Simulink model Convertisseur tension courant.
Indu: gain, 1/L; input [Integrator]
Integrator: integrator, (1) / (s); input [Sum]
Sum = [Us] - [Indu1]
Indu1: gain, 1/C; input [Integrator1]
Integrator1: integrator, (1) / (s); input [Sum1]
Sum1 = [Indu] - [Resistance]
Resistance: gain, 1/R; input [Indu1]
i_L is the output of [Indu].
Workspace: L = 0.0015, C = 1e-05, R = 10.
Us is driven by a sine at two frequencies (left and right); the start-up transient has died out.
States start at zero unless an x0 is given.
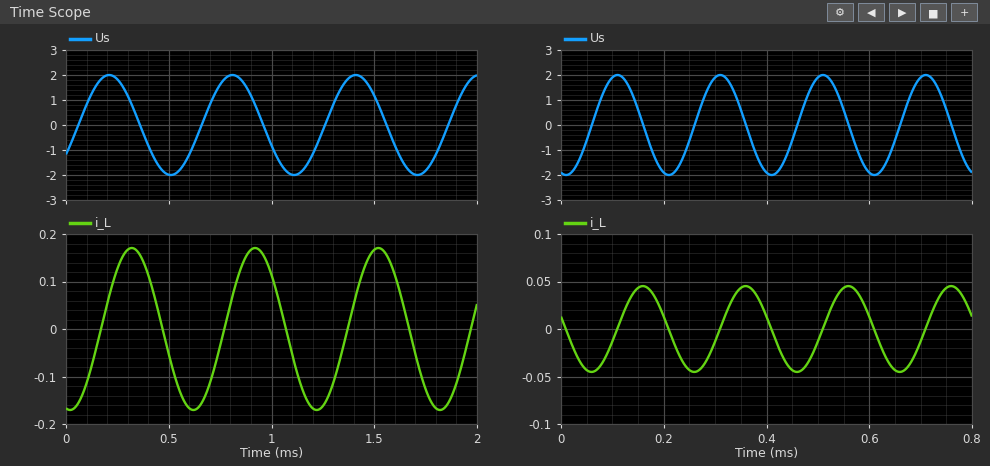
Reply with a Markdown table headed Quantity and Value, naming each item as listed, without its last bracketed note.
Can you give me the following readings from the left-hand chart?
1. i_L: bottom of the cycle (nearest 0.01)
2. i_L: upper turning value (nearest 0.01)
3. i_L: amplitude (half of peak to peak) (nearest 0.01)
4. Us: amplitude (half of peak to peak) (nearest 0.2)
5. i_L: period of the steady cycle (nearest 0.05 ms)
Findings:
| Quantity | Value |
|---|---|
| i_L: bottom of the cycle | -0.17 |
| i_L: upper turning value | 0.17 |
| i_L: amplitude (half of peak to peak) | 0.17 |
| Us: amplitude (half of peak to peak) | 2.0 |
| i_L: period of the steady cycle | 0.60 ms |
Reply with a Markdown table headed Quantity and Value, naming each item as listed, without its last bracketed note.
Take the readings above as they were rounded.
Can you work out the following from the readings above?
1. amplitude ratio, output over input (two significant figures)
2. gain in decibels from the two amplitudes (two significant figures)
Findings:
| Quantity | Value |
|---|---|
| amplitude ratio, output over input | 0.085 |
| gain in decibels from the two amplitudes | -21 dB |
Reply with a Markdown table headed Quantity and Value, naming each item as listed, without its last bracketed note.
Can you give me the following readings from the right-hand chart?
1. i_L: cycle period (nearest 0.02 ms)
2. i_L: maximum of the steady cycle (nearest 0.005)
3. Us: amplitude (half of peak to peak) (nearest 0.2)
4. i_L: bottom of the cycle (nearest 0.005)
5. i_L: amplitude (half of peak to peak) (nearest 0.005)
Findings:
| Quantity | Value |
|---|---|
| i_L: cycle period | 0.20 ms |
| i_L: maximum of the steady cycle | 0.045 |
| Us: amplitude (half of peak to peak) | 2.0 |
| i_L: bottom of the cycle | -0.045 |
| i_L: amplitude (half of peak to peak) | 0.045 |
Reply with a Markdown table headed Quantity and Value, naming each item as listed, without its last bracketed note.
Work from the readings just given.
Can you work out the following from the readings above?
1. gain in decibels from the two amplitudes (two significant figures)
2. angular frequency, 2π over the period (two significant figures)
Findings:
| Quantity | Value |
|---|---|
| gain in decibels from the two amplitudes | -33 dB |
| angular frequency, 2π over the period | 31 rad/ms |
